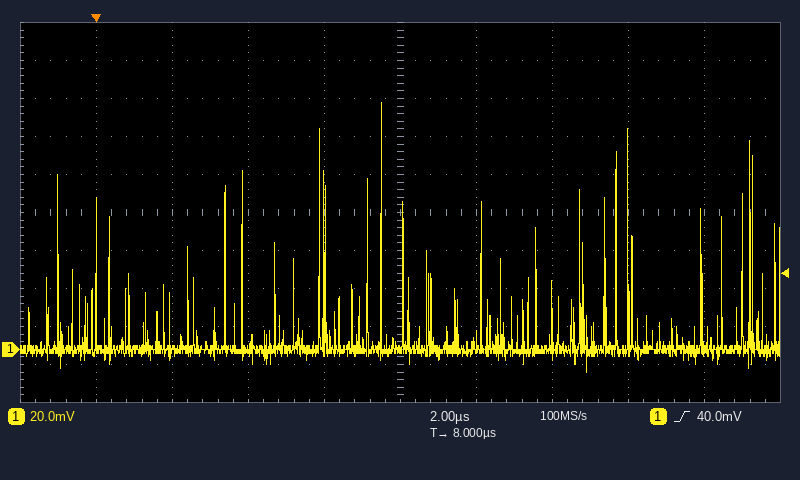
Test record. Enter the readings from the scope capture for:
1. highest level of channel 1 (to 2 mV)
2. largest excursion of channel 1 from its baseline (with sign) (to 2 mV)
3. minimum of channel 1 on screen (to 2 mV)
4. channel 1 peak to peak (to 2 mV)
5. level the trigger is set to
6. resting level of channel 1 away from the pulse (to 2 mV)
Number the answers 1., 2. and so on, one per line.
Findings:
1. 130 mV
2. +130 mV
3. -12 mV
4. 142 mV
5. 40.0 mV
6. 0 mV
